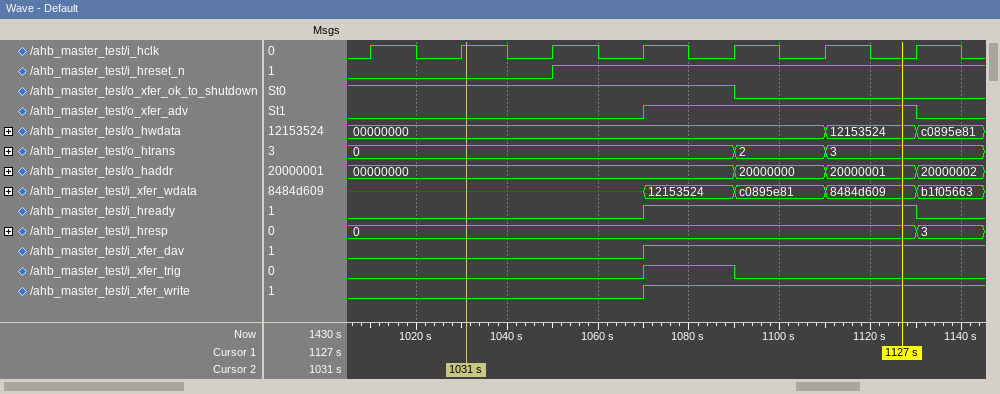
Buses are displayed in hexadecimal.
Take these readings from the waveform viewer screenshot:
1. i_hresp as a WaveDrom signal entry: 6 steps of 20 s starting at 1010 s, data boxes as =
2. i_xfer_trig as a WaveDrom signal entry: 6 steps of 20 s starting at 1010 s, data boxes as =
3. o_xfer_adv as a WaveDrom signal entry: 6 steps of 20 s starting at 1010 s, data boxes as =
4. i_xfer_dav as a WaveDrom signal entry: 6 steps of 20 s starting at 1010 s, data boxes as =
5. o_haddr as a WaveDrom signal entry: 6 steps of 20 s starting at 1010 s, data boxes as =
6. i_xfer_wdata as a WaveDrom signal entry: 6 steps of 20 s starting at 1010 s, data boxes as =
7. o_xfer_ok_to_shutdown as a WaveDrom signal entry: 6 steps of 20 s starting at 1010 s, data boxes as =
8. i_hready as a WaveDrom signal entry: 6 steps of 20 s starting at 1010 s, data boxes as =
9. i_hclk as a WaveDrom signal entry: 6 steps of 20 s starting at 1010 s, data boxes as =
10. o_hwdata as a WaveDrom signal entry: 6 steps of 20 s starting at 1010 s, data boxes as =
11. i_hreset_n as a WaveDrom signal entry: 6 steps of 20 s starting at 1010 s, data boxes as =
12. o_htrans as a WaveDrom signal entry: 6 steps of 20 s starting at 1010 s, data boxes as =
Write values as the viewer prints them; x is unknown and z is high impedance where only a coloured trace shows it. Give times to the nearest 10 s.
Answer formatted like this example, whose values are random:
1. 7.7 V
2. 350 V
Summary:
1. {name: 'i_hresp', wave: '=.....', data: '0'}
2. {name: 'i_xfer_trig', wave: '0..10.'}
3. {name: 'o_xfer_adv', wave: '0..1..'}
4. {name: 'i_xfer_dav', wave: '0..1..'}
5. {name: 'o_haddr', wave: '=...==', data: '00000000 20000000 20000001'}
6. {name: 'i_xfer_wdata', wave: 'x..===', data: '12153524 c0895e81 8484d609'}
7. {name: 'o_xfer_ok_to_shutdown', wave: '1...0.'}
8. {name: 'i_hready', wave: '0..1..'}
9. {name: 'i_hclk', wave: 'p.....'}
10. {name: 'o_hwdata', wave: '=....=', data: '00000000 12153524'}
11. {name: 'i_hreset_n', wave: '0.1...'}
12. {name: 'o_htrans', wave: '=...==', data: '0 2 3'}
